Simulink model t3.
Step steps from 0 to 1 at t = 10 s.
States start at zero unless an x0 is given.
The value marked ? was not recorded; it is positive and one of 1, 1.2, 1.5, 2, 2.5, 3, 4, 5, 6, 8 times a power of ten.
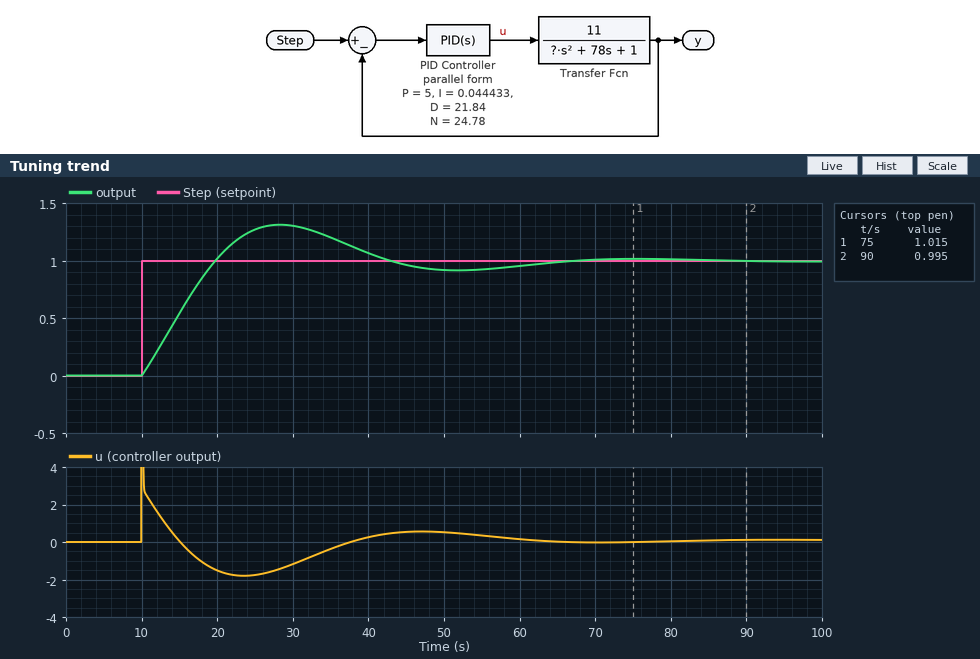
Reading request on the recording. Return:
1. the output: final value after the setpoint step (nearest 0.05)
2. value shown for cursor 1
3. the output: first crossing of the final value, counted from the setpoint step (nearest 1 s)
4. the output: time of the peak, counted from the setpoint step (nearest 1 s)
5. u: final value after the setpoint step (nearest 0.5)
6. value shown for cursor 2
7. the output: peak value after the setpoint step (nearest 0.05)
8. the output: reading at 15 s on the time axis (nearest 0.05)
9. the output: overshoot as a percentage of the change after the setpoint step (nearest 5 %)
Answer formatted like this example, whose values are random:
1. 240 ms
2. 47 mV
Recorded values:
1. 1.00
2. 1.015
3. 10 s
4. 18 s
5. 0.0
6. 0.995
7. 1.30
8. 0.55
9. 30 %
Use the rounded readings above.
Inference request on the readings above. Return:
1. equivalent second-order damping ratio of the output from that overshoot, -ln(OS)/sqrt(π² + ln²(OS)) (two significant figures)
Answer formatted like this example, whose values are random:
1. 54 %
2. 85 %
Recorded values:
1. 0.36
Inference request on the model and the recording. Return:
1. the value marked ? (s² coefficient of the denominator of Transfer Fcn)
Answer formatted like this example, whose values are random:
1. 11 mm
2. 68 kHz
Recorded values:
1. 2500
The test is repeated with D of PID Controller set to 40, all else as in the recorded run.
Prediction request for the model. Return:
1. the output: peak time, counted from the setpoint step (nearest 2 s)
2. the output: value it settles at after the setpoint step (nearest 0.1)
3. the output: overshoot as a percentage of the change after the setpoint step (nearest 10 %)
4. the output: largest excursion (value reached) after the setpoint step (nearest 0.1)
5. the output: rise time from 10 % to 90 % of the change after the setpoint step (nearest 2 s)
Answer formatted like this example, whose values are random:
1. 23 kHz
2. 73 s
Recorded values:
1. 16 s
2. 1.0
3. 20 %
4. 1.2
5. 6 s
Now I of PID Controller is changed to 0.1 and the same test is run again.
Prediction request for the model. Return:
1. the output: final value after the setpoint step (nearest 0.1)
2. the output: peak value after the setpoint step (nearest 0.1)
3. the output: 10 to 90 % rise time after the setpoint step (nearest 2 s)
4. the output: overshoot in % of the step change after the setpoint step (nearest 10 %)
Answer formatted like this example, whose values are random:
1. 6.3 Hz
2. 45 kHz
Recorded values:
1. 1.0
2. 1.4
3. 8 s
4. 40 %
